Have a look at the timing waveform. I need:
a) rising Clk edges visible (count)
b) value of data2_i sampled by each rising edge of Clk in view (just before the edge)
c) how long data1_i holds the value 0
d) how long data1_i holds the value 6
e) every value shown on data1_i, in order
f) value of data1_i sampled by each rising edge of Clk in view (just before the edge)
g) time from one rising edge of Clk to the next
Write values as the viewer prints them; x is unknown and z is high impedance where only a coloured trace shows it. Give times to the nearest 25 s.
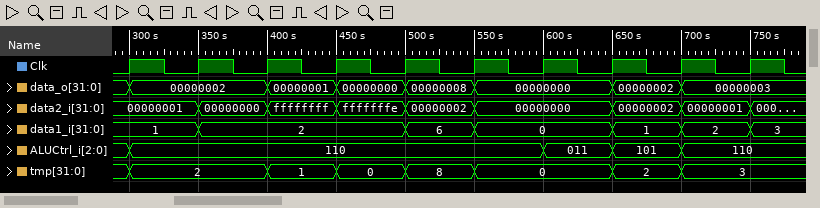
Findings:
10
00000001, 00000001, 00000000, ffffffff, fffffffe, 00000002, 00000000, 00000000, 00000002, 00000001
100 s
50 s
1, 2, 6, 0, 1, 2, 3
1, 1, 2, 2, 2, 6, 0, 0, 1, 2
50 s
